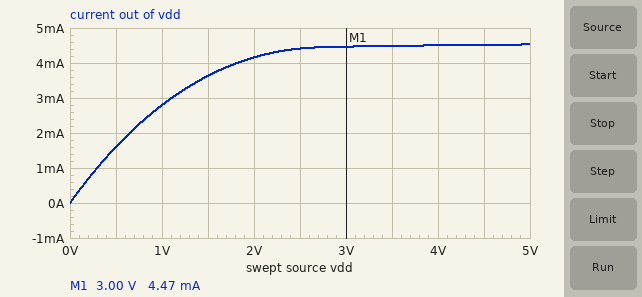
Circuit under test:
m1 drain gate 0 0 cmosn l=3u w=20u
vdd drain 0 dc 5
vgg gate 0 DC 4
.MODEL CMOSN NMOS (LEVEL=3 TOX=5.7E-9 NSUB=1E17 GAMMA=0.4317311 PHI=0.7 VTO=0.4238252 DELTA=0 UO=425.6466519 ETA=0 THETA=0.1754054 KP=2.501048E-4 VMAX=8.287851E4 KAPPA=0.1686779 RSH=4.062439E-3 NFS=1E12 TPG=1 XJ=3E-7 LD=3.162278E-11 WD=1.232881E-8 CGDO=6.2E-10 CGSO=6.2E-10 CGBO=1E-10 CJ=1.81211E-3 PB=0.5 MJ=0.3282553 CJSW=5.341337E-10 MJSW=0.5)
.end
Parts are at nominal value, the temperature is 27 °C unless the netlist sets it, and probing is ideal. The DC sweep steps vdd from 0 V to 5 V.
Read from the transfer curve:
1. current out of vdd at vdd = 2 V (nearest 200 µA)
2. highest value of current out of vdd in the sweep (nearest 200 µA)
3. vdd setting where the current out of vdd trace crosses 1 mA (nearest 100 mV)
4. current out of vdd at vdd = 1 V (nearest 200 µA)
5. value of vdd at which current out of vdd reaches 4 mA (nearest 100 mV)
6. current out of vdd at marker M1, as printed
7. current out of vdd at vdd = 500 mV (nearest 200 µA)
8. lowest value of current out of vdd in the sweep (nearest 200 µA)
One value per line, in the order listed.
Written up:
4.2 mA
4.6 mA
300 mV
2.8 mA
1.8 V
4.47 mA
1.6 mA
0 A
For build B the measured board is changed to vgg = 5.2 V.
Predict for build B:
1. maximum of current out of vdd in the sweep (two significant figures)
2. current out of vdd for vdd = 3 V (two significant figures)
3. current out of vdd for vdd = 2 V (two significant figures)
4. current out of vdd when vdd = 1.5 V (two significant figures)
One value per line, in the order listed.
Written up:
6.8 mA
6.6 mA
5.6 mA
4.7 mA
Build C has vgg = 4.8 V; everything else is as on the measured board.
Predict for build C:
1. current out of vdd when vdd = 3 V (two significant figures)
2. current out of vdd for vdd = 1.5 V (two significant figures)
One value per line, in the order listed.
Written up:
5.9 mA
4.4 mA
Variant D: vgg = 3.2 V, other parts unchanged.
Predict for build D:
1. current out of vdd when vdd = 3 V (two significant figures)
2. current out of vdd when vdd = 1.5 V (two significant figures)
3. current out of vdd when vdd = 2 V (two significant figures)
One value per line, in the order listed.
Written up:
3.1 mA
2.8 mA
3.0 mA
